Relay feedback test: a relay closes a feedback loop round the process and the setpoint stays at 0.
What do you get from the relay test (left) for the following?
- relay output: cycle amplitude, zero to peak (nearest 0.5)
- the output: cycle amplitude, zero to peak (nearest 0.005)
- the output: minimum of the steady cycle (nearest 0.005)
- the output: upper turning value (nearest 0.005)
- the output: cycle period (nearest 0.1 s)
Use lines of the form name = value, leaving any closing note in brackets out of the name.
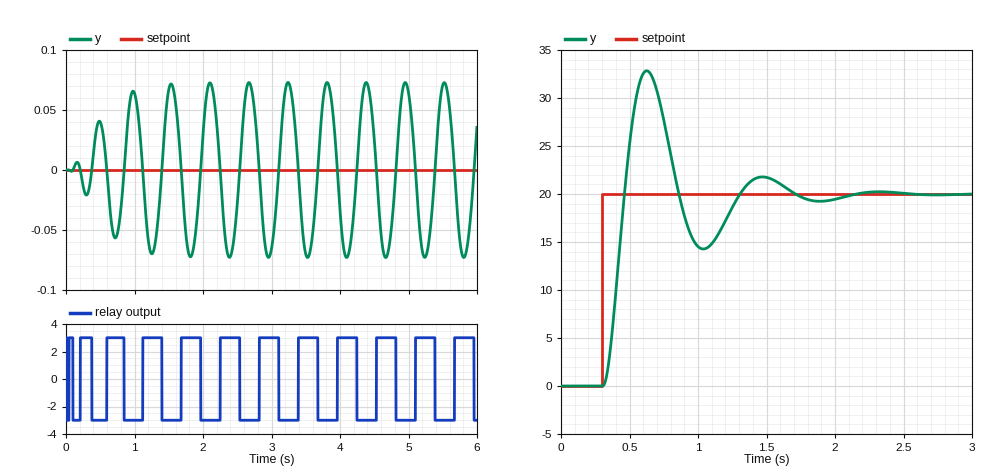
relay output: cycle amplitude, zero to peak = 3.0
the output: cycle amplitude, zero to peak = 0.075
the output: minimum of the steady cycle = -0.075
the output: upper turning value = 0.075
the output: cycle period = 0.6 s
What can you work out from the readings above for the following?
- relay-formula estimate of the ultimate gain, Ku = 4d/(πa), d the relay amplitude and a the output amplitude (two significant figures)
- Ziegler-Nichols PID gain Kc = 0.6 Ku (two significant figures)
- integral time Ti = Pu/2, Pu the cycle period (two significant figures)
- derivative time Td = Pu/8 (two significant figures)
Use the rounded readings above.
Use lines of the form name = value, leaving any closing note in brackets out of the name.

relay-formula estimate of the ultimate gain, Ku = 4d/(πa), d the relay amplitude and a the output amplitude = 51
Ziegler-Nichols PID gain Kc = 0.6 Ku = 31
integral time Ti = Pu/2, Pu the cycle period = 0.30 s
derivative time Td = Pu/8 = 0.075 s
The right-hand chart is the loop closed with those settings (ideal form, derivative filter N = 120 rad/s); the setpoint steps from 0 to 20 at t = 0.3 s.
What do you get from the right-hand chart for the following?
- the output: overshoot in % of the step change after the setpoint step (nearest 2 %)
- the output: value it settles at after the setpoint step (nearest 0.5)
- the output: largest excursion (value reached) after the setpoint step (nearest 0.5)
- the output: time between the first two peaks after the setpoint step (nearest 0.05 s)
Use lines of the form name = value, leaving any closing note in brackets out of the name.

the output: overshoot in % of the step change after the setpoint step = 64 %
the output: value it settles at after the setpoint step = 20.0
the output: largest excursion (value reached) after the setpoint step = 33.0
the output: time between the first two peaks after the setpoint step = 0.85 s
